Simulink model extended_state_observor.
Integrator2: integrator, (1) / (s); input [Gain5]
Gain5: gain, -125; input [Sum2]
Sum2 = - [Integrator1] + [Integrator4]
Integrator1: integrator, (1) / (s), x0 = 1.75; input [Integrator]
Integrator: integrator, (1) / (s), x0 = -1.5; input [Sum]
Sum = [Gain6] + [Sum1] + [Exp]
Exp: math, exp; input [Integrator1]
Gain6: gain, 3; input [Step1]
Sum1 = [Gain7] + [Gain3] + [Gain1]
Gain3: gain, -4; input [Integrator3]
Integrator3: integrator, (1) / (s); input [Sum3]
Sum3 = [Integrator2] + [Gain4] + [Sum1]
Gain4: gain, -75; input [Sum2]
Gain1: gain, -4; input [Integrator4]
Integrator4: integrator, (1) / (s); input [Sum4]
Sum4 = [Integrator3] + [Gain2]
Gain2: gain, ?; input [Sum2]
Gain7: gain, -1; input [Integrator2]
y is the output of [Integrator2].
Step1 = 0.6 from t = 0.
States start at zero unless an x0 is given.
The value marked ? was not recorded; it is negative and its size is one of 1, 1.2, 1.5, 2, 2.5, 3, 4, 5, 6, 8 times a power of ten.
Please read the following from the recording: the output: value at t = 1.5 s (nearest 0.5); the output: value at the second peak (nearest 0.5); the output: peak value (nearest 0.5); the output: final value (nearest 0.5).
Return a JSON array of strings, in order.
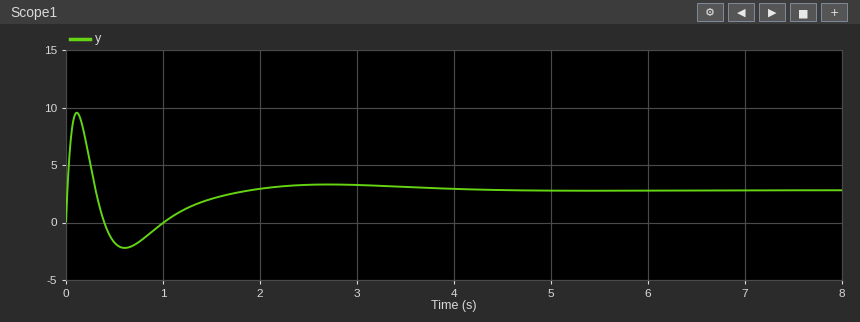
["2.0", "3.5", "9.5", "3.0"]
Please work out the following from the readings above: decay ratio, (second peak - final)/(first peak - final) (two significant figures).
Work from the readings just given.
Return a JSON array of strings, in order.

["0.077"]
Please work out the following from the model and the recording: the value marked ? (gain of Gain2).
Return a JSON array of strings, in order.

["-15"]
